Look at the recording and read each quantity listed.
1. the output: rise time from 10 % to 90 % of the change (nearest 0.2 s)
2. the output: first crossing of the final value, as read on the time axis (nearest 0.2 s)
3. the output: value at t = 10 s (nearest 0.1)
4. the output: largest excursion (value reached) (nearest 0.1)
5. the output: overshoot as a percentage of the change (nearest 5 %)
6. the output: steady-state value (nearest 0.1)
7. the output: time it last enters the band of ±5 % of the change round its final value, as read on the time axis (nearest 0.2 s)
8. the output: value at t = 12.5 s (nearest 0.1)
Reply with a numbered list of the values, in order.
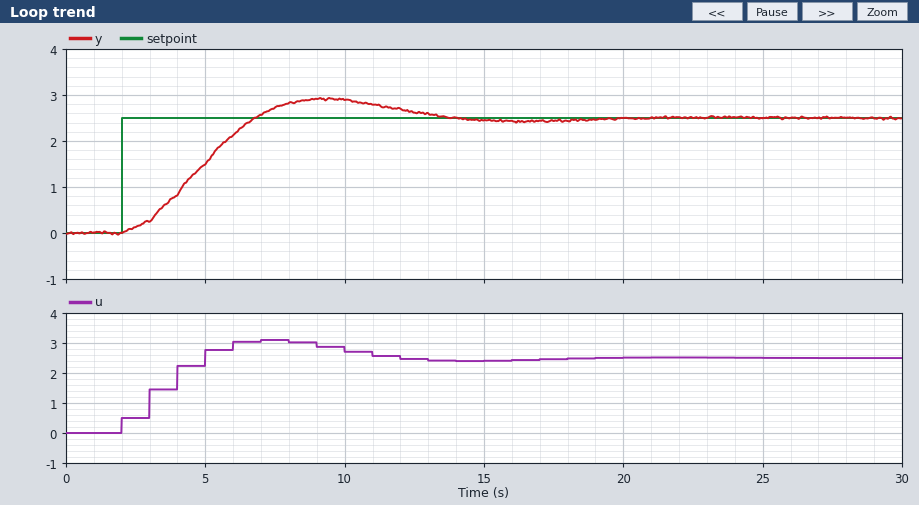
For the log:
1. 3.2 s
2. 6.8 s
3. 2.9
4. 2.9
5. 15 %
6. 2.5
7. 12.6 s
8. 2.6
